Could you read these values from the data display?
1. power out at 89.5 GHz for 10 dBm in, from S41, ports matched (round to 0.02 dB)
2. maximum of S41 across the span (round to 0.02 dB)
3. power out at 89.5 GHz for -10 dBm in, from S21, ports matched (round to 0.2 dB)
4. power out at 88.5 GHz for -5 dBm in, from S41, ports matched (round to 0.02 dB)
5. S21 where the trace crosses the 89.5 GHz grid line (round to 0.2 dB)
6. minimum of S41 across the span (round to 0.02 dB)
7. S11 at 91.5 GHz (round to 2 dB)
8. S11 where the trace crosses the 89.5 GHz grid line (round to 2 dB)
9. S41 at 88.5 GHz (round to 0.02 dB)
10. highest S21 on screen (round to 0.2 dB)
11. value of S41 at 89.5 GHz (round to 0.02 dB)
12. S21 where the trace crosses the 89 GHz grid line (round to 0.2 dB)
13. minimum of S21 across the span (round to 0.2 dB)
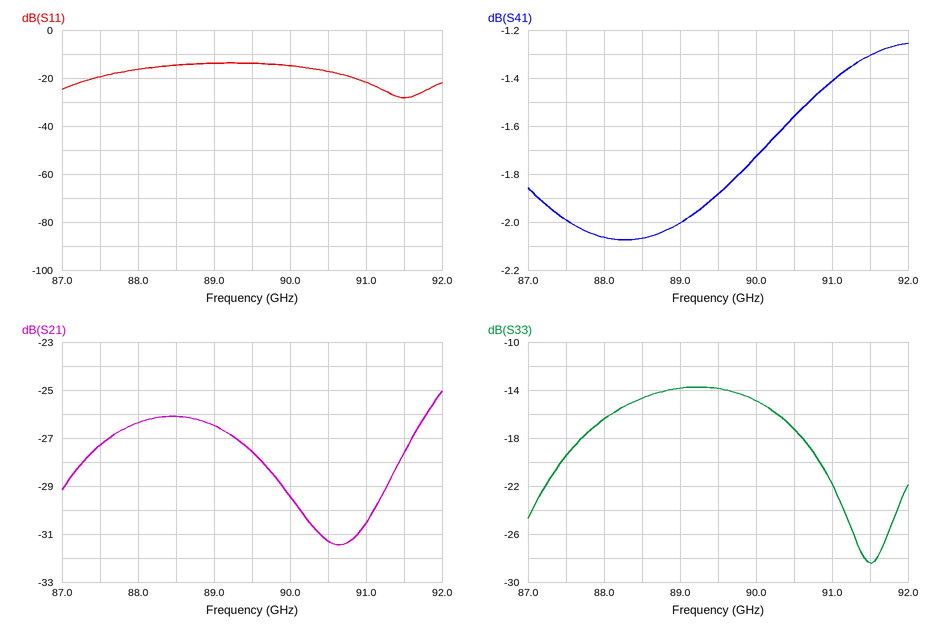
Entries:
8.12 dBm
-1.26 dB
-37.6 dBm
-7.06 dBm
-27.6 dB
-2.08 dB
-28 dB
-14 dB
-2.06 dB
-25.0 dB
-1.88 dB
-26.4 dB
-31.4 dB
